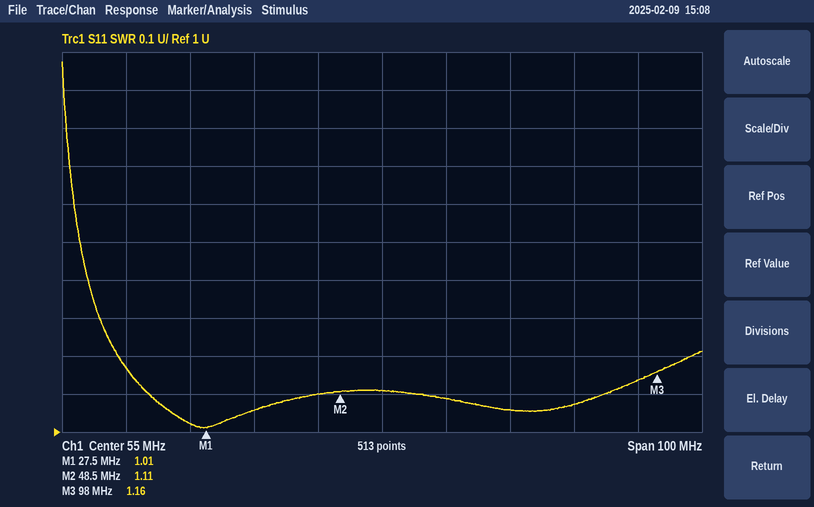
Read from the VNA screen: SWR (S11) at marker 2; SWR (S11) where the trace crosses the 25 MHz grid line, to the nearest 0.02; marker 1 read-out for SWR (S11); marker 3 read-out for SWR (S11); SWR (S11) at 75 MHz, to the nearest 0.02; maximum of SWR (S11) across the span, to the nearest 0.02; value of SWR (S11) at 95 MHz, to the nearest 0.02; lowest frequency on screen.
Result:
1.11
1.02
1.01
1.16
1.06
1.98
1.14
5 MHz
